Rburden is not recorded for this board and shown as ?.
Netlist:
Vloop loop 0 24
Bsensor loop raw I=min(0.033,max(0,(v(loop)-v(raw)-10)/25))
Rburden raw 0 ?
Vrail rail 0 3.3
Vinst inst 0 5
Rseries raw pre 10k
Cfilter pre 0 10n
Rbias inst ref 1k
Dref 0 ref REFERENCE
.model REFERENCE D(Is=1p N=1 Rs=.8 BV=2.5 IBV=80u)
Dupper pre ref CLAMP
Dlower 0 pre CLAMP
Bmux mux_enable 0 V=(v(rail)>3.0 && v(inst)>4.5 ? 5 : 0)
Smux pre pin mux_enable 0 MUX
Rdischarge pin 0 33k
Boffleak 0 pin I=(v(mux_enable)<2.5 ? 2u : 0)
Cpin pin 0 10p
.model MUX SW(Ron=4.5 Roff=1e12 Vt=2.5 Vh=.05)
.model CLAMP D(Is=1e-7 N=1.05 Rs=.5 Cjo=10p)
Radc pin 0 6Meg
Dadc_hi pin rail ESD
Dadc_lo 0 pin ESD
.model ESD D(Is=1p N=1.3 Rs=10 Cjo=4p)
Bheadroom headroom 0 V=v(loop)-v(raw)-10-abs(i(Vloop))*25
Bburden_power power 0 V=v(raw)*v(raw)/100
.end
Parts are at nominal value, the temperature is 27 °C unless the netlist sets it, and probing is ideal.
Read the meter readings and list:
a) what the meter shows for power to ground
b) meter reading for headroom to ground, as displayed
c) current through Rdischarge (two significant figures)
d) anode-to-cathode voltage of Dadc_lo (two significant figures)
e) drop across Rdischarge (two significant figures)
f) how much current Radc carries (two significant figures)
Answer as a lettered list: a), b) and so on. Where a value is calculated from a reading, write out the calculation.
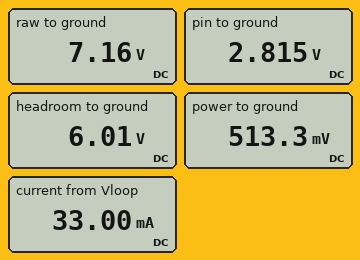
a) 513.3 mV
b) 6.01 V
c) (2.815 V) / 33 kΩ = 85 µA
d) 0 V - 2.815 V = -2.8 V
e) 2.815 V = 2.8 V
f) (2.815 V) / 6 MΩ = 470 nA
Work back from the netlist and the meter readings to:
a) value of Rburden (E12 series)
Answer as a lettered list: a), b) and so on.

a) 220 Ω
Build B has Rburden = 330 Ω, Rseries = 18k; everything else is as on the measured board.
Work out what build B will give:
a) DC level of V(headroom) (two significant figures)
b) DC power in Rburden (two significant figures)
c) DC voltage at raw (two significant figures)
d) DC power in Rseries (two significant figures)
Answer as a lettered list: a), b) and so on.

a) 2.4 V
b) 350 mW
c) 11 V
d) 3.5 mW
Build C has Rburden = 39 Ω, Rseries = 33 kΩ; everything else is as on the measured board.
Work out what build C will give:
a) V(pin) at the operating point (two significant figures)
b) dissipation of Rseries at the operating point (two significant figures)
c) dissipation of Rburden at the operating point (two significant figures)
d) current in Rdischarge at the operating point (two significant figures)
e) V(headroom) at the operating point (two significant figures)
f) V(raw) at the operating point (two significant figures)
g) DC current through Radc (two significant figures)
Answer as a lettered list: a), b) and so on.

a) 640 mV
b) 13 µW
c) 42 mW
d) 19 µA
e) 12 V
f) 1.3 V
g) 110 nA
